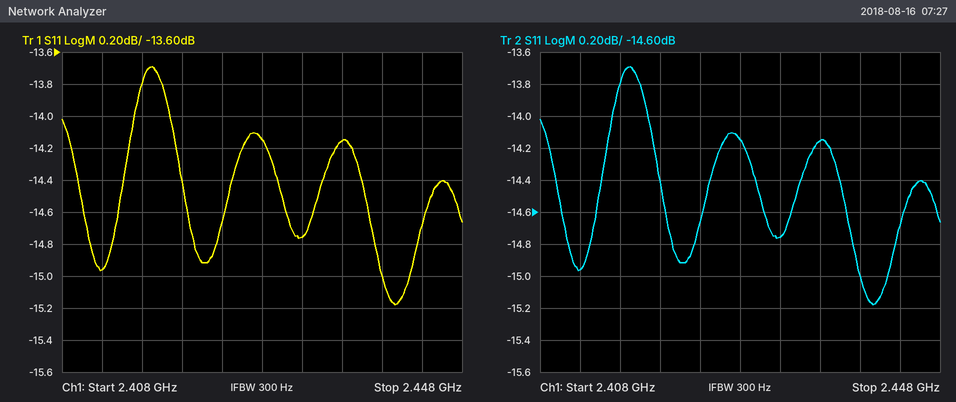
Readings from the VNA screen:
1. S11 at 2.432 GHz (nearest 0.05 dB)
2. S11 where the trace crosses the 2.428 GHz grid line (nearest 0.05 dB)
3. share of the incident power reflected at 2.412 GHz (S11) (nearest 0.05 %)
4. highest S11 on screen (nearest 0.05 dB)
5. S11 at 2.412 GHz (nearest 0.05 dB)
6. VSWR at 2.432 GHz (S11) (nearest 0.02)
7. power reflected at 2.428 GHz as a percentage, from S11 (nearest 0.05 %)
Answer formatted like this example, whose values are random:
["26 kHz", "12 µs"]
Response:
["-14.75 dB", "-14.15 dB", "3.20 %", "-13.70 dB", "-14.95 dB", "1.44", "3.85 %"]
